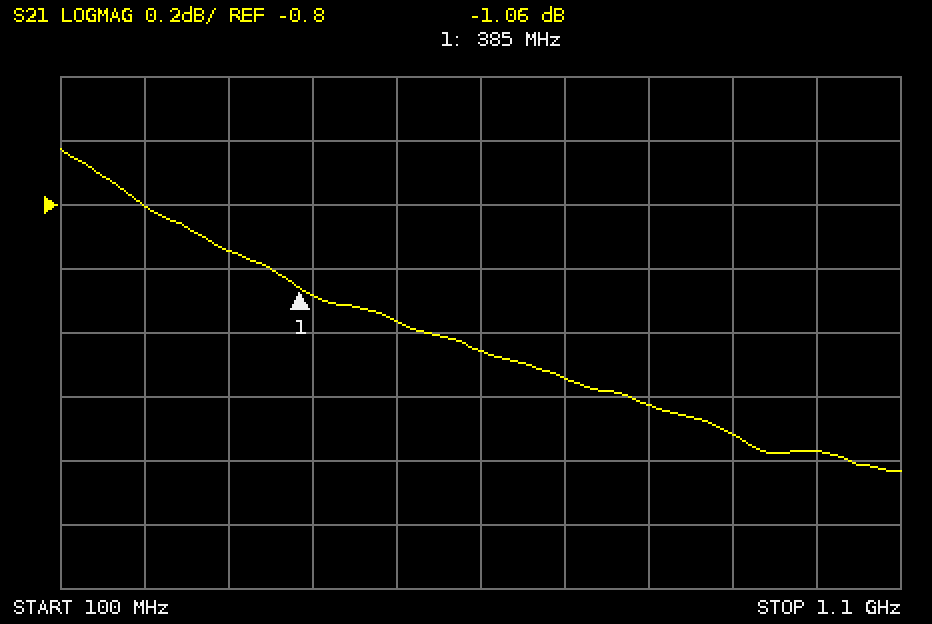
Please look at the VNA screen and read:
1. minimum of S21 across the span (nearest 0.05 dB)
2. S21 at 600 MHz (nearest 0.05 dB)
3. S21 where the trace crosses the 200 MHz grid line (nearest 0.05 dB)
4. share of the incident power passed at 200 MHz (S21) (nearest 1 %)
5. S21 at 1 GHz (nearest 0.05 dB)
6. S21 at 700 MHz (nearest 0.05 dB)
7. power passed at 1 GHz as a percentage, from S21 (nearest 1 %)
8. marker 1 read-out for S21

-1.65 dB
-1.25 dB
-0.80 dB
83 %
-1.55 dB
-1.35 dB
70 %
-1.06 dB
